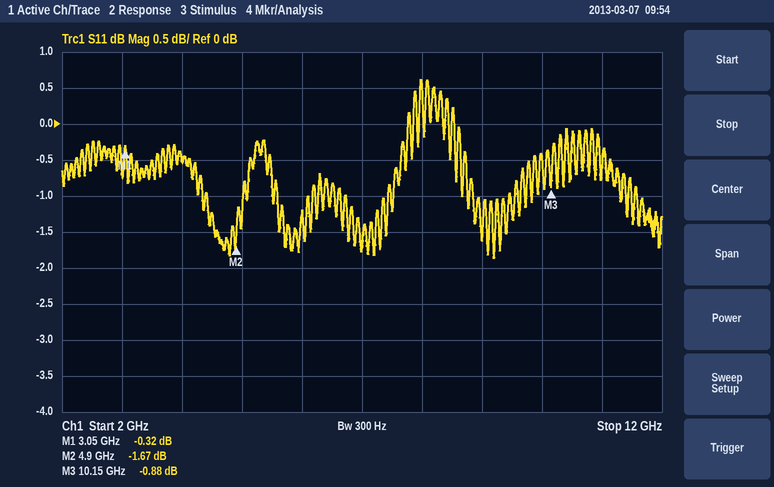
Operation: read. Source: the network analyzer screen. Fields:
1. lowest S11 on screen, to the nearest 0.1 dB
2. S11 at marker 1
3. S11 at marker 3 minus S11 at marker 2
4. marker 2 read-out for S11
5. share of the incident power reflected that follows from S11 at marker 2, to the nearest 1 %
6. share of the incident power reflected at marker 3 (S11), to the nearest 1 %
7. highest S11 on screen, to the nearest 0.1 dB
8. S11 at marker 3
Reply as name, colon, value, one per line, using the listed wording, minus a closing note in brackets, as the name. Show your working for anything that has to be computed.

lowest S11 on screen, to the nearest 0.1 dB: -1.9 dB
S11 at marker 1: -0.32 dB
S11 at marker 3 minus S11 at marker 2: -0.88 − (-1.67) = 0.79 dB
marker 2 read-out for S11: -1.67 dB
share of the incident power reflected that follows from S11 at marker 2, to the nearest 1 %: 10^(-1.67/10) ≈ 68 %
share of the incident power reflected at marker 3 (S11), to the nearest 1 %: 10^(-0.88/10) ≈ 82 %
highest S11 on screen, to the nearest 0.1 dB: 0.6 dB
S11 at marker 3: -0.88 dB
